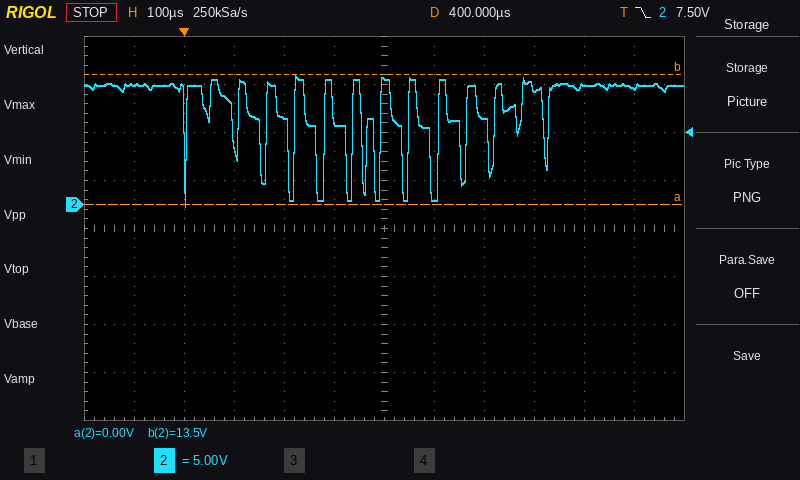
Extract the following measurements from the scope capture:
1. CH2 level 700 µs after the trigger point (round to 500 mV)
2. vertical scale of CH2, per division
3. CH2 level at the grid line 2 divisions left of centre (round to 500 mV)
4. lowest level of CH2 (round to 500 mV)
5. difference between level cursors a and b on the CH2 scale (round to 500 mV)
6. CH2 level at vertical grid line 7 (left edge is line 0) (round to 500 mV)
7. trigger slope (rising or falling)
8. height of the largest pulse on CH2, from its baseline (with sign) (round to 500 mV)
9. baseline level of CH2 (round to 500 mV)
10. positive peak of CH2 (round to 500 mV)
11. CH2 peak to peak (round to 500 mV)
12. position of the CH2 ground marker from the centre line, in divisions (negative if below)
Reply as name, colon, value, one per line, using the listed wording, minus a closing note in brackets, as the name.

CH2 level 700 µs after the trigger point: 12.5 V
vertical scale of CH2, per division: 5 V
CH2 level at the grid line 2 divisions left of centre: 9.0 V
lowest level of CH2: 0.0 V
difference between level cursors a and b on the CH2 scale: 13.5 V
CH2 level at vertical grid line 7 (left edge is line 0): 1.0 V
trigger slope: falling
height of the largest pulse on CH2, from its baseline (with sign): -12.5 V
baseline level of CH2: 12.5 V
positive peak of CH2: 13.5 V
CH2 peak to peak: 13.5 V
position of the CH2 ground marker from the centre line, in divisions: +0.5 div
